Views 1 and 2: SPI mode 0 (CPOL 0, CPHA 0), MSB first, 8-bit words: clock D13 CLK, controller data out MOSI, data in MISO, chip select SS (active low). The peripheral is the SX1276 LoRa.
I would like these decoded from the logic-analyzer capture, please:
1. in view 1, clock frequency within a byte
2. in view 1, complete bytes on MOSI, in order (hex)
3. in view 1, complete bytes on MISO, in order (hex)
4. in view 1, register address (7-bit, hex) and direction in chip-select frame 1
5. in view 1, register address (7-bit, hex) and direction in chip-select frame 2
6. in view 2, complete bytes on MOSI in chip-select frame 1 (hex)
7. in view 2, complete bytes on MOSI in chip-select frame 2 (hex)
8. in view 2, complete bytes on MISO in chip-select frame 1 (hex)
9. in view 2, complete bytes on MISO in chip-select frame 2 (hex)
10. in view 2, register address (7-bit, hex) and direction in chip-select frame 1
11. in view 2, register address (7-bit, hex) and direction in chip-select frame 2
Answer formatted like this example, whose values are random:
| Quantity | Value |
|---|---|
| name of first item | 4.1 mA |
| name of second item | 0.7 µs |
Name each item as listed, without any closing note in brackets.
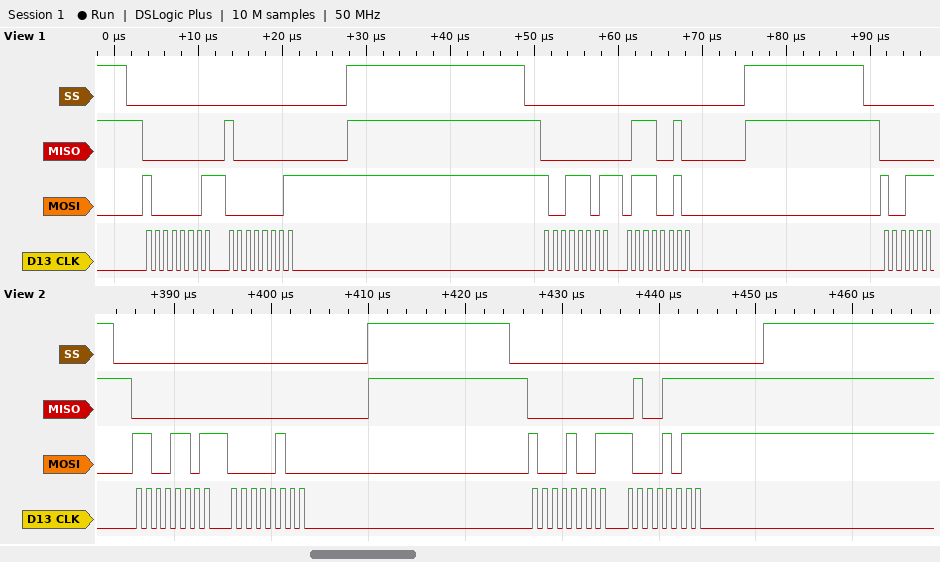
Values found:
| Quantity | Value |
|---|---|
| in view 1, clock frequency within a byte | 1 MHz |
| in view 1, complete bytes on MOSI, in order | 81 01 9D 72 |
| in view 1, complete bytes on MISO, in order | 00 80 00 72 |
| in view 1, register address (7-bit, hex) and direction in chip-select frame 1 | 0x01 write |
| in view 1, register address (7-bit, hex) and direction in chip-select frame 2 | 0x1D write |
| in view 2, complete bytes on MOSI in chip-select frame 1 | CD 04 |
| in view 2, complete bytes on MOSI in chip-select frame 2 | 89 8B |
| in view 2, complete bytes on MISO in chip-select frame 1 | 00 00 |
| in view 2, complete bytes on MISO in chip-select frame 2 | 00 4F |
| in view 2, register address (7-bit, hex) and direction in chip-select frame 1 | 0x4D write |
| in view 2, register address (7-bit, hex) and direction in chip-select frame 2 | 0x09 write |
